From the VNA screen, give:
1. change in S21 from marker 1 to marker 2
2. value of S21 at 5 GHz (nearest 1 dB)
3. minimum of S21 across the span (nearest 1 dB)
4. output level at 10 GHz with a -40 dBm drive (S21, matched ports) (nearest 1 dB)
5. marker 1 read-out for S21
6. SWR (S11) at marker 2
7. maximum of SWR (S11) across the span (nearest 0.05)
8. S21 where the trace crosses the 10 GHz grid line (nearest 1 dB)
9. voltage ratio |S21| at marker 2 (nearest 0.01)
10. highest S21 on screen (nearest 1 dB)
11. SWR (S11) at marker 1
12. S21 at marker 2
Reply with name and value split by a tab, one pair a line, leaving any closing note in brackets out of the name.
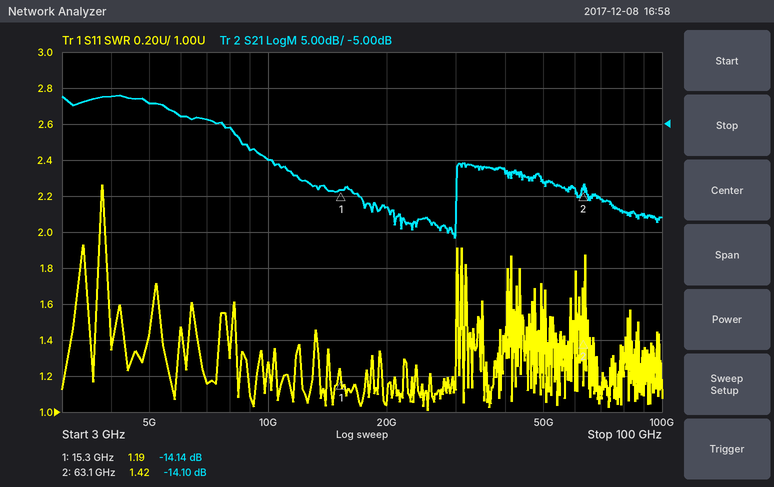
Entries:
change in S21 from marker 1 to marker 2	0.04 dB
value of S21 at 5 GHz	-2 dB
minimum of S21 across the span	-21 dB
output level at 10 GHz with a -40 dBm drive (S21, matched ports)	-50 dBm
marker 1 read-out for S21	-14.14 dB
SWR (S11) at marker 2	1.42
maximum of SWR (S11) across the span	2.25
S21 where the trace crosses the 10 GHz grid line	-10 dB
voltage ratio |S21| at marker 2	0.20
highest S21 on screen	-1 dB
SWR (S11) at marker 1	1.19
S21 at marker 2	-14.10 dB
